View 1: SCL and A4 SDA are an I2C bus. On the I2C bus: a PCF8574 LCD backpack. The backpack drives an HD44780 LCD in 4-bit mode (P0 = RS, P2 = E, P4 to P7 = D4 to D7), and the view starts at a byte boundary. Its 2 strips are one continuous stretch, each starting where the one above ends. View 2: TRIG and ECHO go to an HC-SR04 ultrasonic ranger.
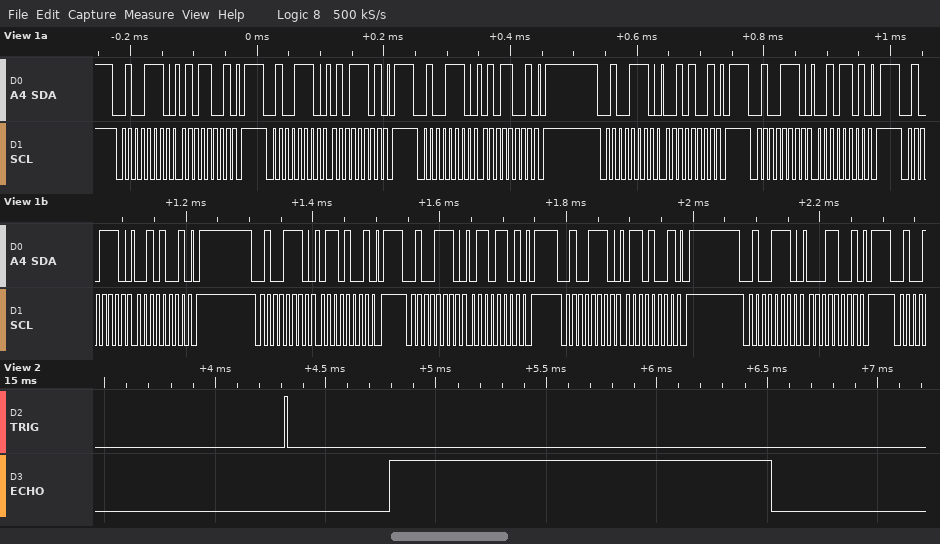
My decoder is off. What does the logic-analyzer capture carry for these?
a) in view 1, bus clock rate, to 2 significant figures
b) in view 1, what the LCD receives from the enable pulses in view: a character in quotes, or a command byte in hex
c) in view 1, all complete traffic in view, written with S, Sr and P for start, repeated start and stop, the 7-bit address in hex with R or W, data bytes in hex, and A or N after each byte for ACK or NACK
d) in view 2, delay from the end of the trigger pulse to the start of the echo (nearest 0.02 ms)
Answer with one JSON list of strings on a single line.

["100 kHz", "'R'", "S 27W A 59 A P S 27W A 5D A P S 27W A 59 A P S 27W A 29 A P S 27W A 2D A P S 27W A 29 A P S 27W A 69 A P S 27W A 6D A P S 27W A 69 A P S 27W A 19 A P", "0.46 ms"]
